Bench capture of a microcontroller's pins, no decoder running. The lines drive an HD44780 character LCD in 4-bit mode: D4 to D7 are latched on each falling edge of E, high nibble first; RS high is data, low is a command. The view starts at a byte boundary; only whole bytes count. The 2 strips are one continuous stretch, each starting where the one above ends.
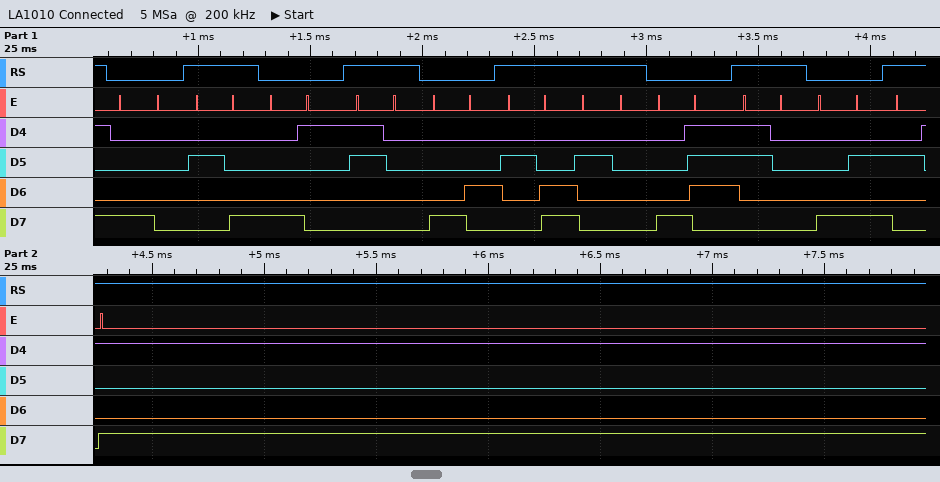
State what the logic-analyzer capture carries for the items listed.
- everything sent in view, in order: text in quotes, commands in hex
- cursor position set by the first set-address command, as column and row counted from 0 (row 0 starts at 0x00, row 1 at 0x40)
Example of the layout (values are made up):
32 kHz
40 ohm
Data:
0x80 "(" 0x81 "0" 0x84 ", " 0x87 "0" 0x8A ")"
column 0, row 0
